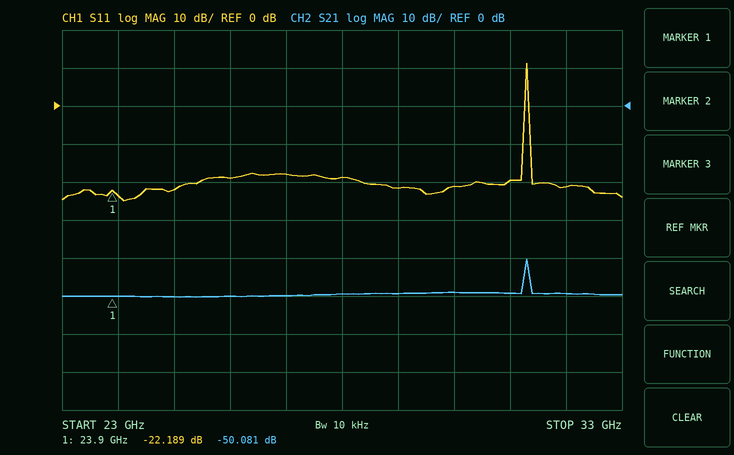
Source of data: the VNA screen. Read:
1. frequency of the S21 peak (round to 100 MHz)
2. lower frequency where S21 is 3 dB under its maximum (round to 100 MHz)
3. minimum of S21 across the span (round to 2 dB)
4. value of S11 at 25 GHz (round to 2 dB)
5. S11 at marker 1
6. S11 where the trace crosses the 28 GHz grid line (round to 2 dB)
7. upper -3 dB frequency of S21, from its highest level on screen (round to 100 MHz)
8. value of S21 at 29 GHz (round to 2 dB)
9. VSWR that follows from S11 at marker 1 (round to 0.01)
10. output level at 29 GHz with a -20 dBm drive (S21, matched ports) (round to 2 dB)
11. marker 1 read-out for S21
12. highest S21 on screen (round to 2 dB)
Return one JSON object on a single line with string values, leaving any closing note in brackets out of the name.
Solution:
{"frequency of the S21 peak": "31.3 GHz", "lower frequency where S21 is 3 dB under its maximum": "31.3 GHz", "minimum of S21 across the span": "-50 dB", "value of S11 at 25 GHz": "-22 dB", "S11 at marker 1": "-22.189 dB", "S11 where the trace crosses the 28 GHz grid line": "-18 dB", "upper -3 dB frequency of S21, from its highest level on screen": "31.3 GHz", "value of S21 at 29 GHz": "-50 dB", "VSWR that follows from S11 at marker 1": "1.17", "output level at 29 GHz with a -20 dBm drive (S21, matched ports)": "-70 dBm", "marker 1 read-out for S21": "-50.081 dB", "highest S21 on screen": "-40 dB"}
